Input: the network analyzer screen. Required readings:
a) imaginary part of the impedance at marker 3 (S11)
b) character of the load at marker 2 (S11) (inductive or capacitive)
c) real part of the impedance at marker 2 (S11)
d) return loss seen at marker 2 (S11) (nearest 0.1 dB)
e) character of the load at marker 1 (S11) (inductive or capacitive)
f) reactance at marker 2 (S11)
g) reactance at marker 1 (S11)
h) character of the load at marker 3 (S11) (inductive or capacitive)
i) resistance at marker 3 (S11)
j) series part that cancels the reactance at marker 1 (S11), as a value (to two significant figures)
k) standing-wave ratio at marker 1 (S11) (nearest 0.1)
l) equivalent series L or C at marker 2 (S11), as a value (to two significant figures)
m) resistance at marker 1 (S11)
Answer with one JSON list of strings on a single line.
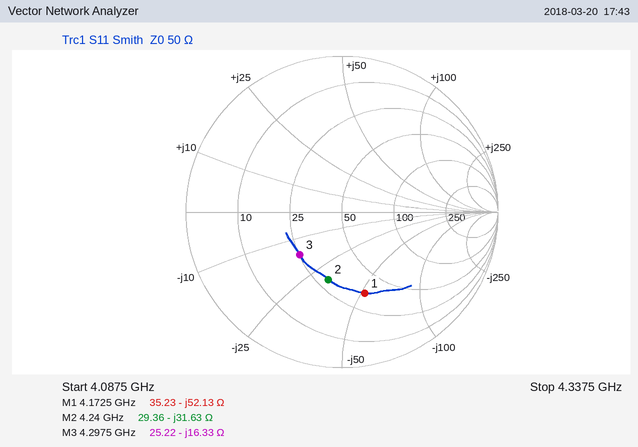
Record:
["-16.33 Ω", "capacitive", "29.36 Ω", "7.1 dB", "capacitive", "-31.63 Ω", "-52.13 Ω", "capacitive", "25.22 Ω", "2.0 nH", "3.4", "1.2 pF", "35.23 Ω"]
